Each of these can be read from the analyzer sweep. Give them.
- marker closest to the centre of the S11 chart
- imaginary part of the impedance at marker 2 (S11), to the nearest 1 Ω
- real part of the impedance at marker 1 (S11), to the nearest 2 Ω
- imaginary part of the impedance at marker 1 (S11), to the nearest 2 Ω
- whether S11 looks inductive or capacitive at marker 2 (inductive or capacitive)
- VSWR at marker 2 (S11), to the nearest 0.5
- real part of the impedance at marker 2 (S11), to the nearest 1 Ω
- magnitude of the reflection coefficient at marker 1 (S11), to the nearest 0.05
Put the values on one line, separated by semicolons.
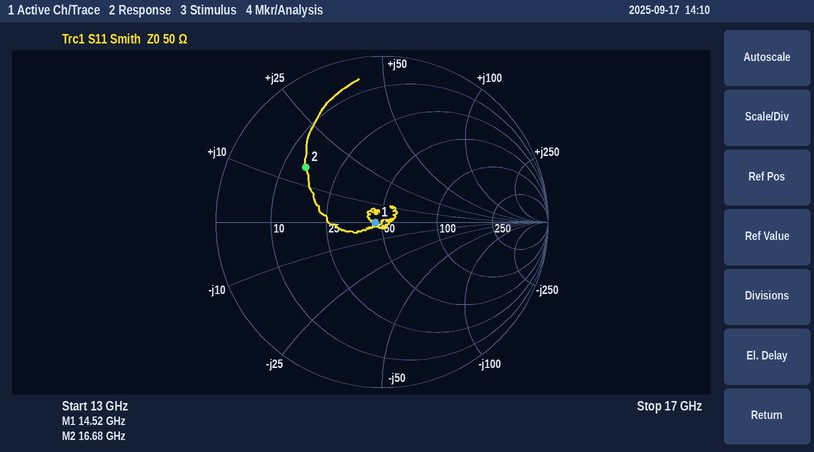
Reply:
marker 1; +15 Ω; 46 Ω; 0 Ω; inductive; 3.5; 15 Ω; 0.05
